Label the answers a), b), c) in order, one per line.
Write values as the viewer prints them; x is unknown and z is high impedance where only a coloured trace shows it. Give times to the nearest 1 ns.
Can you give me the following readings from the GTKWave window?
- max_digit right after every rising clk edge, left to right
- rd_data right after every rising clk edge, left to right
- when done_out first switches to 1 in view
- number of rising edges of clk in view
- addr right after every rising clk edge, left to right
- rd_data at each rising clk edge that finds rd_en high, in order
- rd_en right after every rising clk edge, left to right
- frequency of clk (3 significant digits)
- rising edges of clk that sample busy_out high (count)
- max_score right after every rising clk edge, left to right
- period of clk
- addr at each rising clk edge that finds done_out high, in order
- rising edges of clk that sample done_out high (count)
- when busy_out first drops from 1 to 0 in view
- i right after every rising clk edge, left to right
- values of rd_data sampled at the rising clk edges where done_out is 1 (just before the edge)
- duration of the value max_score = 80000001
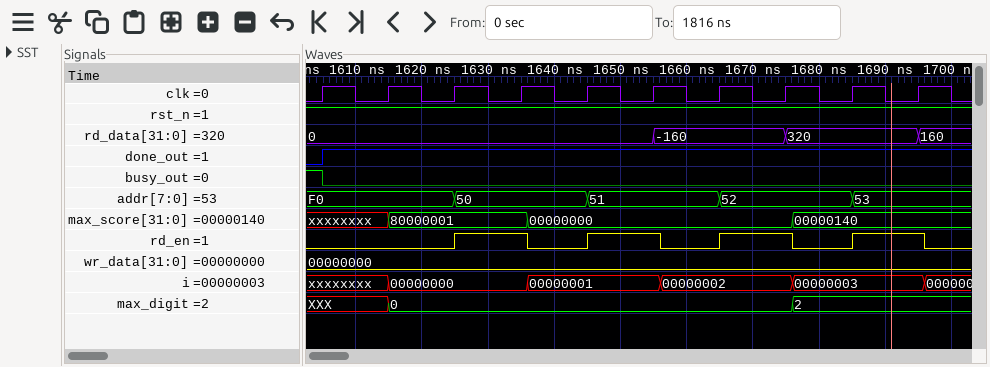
a) XXX, 0, 0, 0, 0, 0, 0, 0, 2, 2
b) 0, 0, 0, 0, 0, -160, -160, 320, 320, 160
c) 1605 ns
d) 10
e) F0, F0, 50, 50, 51, 51, 52, 52, 53, 53
f) 0, 0, -160, 320
g) 0 0 1 1 1 1 1 1 1 1
h) 100 MHz
i) 1
j) xxxxxxxx, 80000001, 80000001, 80000001, 00000000, 00000000, 00000000, 00000000, 00000140, 00000140
k) 10 ns
l) F0, F0, 50, 50, 51, 51, 52, 52, 53
m) 9
n) 1605 ns
o) xxxxxxxx, 00000000, 00000000, 00000000, 00000001, 00000001, 00000002, 00000002, 00000003, 00000003
p) 0, 0, 0, 0, 0, -160, -160, 320, 320
q) 21 ns
